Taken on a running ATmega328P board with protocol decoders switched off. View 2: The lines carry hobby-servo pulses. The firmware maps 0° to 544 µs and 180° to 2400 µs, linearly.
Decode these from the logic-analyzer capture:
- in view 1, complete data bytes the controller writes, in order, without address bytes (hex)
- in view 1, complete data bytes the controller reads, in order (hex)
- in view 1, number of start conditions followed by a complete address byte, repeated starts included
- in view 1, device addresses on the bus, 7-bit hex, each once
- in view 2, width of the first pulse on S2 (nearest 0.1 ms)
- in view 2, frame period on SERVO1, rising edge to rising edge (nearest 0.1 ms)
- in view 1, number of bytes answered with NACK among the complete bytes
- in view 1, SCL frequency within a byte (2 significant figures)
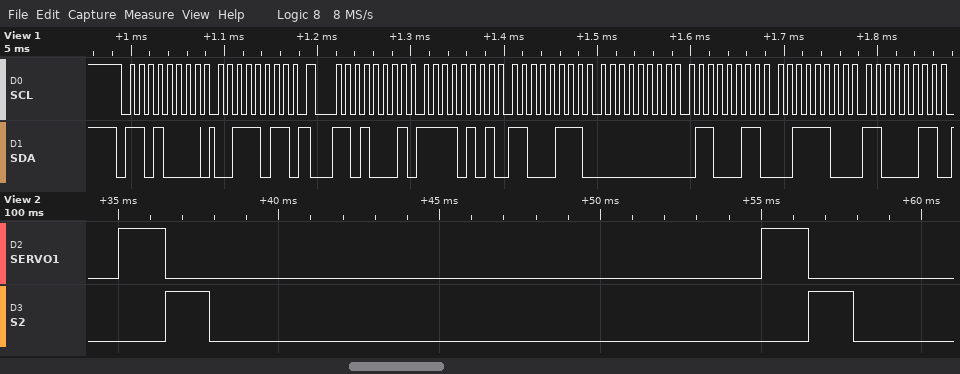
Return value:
3B
F5 C7 00 63 3C C3
2
0x68
1.4 ms
20.0 ms
0
100 kHz
